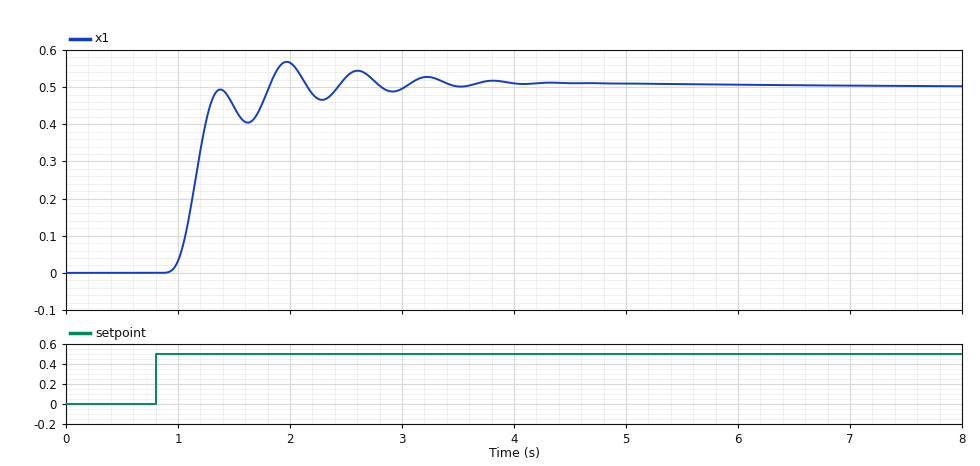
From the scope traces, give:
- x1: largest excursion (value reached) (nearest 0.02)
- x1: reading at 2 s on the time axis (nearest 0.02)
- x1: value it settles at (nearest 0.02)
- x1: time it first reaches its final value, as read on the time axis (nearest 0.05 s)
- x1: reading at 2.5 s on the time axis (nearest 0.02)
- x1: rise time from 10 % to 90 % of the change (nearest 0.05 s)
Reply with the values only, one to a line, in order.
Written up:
0.56
0.56
0.50
1.80 s
0.52
0.25 s
